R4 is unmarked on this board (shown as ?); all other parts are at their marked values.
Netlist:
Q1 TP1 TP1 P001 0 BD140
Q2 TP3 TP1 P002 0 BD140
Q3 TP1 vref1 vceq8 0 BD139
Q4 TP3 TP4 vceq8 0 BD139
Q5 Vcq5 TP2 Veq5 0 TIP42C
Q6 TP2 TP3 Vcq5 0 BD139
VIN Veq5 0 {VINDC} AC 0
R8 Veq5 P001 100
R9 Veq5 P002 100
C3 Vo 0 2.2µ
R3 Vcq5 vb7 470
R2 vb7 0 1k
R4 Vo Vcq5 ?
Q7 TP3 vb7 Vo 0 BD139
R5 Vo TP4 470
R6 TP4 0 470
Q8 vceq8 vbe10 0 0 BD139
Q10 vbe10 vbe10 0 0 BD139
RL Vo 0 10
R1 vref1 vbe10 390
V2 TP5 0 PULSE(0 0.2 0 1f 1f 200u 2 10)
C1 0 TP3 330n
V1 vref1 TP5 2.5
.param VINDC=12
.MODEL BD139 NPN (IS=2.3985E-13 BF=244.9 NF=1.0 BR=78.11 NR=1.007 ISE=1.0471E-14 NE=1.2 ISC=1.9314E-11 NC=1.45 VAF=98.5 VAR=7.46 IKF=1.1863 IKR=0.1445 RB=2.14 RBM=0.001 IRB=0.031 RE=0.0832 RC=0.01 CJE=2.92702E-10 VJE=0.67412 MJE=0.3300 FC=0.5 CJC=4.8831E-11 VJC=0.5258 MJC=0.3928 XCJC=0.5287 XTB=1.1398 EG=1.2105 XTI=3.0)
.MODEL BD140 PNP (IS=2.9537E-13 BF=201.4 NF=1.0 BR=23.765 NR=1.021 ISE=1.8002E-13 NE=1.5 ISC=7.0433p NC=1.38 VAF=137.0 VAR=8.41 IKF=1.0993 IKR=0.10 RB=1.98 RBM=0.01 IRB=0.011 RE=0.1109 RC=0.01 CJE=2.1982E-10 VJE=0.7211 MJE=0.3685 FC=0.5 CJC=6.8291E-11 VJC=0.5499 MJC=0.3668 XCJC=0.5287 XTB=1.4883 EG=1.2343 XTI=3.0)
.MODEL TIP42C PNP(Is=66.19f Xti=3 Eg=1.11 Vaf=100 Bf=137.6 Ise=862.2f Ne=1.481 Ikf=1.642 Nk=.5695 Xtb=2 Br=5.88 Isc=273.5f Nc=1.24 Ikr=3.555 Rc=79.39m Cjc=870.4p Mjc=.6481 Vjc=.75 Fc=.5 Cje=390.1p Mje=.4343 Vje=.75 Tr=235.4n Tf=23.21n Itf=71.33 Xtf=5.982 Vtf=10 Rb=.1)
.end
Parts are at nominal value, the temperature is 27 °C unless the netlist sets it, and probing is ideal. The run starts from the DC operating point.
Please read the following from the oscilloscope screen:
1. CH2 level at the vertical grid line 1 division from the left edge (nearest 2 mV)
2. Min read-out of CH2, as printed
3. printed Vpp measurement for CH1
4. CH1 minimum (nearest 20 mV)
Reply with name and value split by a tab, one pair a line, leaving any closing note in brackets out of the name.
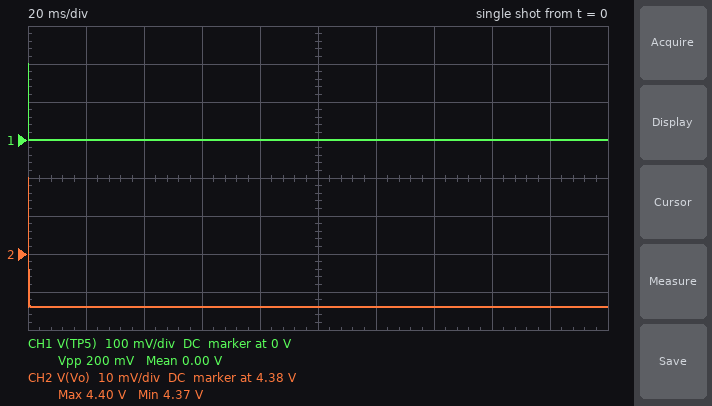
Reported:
CH2 level at the vertical grid line 1 division from the left edge	4.366 V
Min read-out of CH2, as printed	4.37 V
printed Vpp measurement for CH1	200 mV
CH1 minimum	0 V
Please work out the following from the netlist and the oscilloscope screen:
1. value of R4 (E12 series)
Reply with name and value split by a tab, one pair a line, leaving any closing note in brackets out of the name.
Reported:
value of R4	6.8 Ω
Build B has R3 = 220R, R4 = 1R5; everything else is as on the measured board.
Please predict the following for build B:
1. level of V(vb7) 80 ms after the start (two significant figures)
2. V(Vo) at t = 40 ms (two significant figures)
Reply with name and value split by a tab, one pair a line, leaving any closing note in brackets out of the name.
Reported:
level of V(vb7) 80 ms after the start	4.7 V
V(Vo) at t = 40 ms	5.0 V
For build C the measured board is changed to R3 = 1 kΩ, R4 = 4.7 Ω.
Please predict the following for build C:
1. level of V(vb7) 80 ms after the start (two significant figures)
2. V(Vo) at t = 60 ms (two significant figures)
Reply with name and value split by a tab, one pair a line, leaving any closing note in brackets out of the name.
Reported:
level of V(vb7) 80 ms after the start	3.7 V
V(Vo) at t = 60 ms	5.0 V
